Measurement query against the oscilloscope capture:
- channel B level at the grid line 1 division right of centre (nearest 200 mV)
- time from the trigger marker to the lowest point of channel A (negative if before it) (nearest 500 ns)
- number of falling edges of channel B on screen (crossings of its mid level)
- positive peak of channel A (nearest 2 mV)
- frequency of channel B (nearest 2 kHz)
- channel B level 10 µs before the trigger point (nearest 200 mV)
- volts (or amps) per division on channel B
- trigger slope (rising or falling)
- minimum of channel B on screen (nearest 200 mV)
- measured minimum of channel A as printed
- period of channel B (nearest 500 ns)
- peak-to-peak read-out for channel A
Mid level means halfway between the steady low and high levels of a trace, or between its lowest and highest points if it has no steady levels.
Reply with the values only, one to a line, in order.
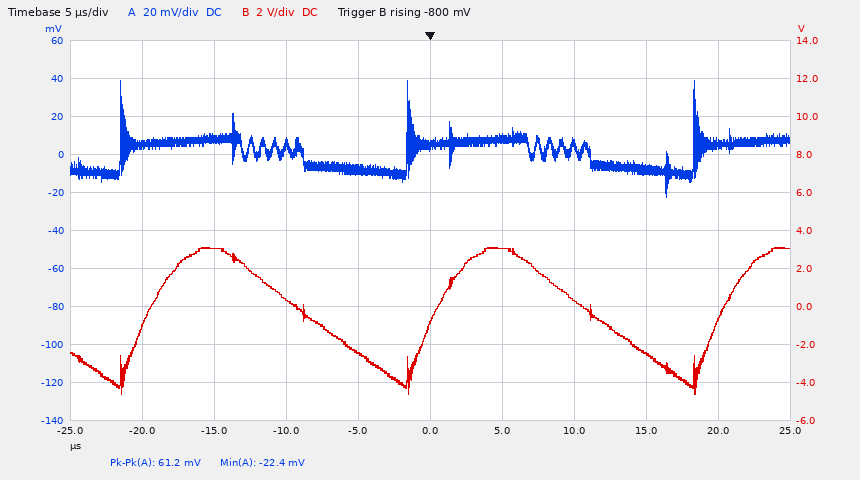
3.0 V
+16.5 µs
2
38 mV
50 kHz
400 mV
2 V
rising
-4.6 V
-22.4 mV
20.0 µs
61.2 mV
